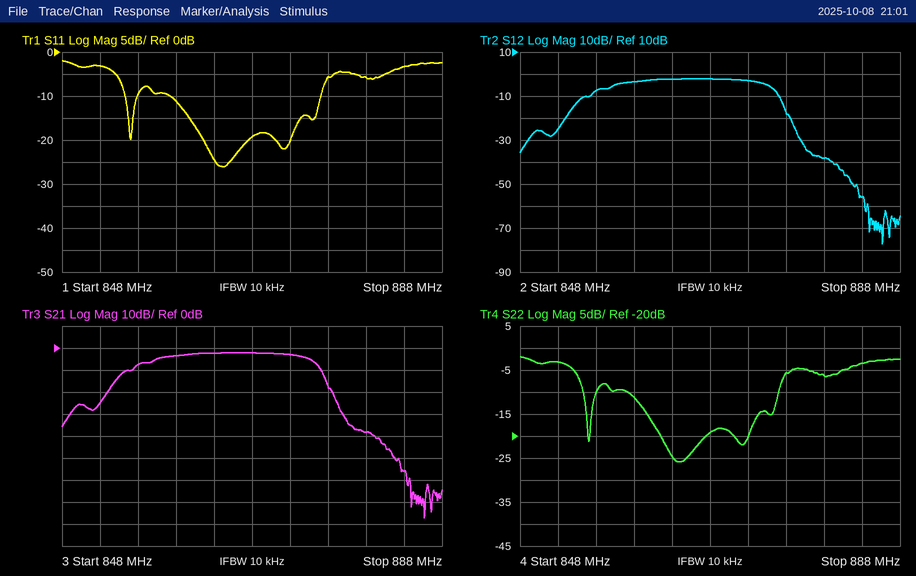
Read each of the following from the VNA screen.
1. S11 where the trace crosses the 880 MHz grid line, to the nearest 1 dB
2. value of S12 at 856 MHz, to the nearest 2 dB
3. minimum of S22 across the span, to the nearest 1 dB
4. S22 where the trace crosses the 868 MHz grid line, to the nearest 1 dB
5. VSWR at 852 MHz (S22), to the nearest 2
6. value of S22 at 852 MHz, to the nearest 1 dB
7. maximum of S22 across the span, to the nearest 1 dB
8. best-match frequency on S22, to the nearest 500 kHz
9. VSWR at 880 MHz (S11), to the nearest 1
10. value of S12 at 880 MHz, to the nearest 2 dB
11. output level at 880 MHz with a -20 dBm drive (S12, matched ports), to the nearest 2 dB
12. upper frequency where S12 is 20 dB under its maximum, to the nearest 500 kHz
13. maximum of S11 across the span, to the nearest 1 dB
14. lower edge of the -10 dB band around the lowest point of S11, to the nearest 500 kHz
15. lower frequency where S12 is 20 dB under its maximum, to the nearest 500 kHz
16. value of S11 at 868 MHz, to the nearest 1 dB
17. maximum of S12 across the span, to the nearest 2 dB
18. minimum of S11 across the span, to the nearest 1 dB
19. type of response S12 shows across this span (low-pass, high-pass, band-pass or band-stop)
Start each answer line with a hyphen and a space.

- -6 dB
- -8 dB
- -26 dB
- -19 dB
- 6
- -3 dB
- -2 dB
- 864.5 MHz
- 3
- -38 dB
- -58 dBm
- 876.5 MHz
- -2 dB
- 859.5 MHz
- 852.5 MHz
- -19 dB
- -2 dB
- -26 dB
- band-pass
